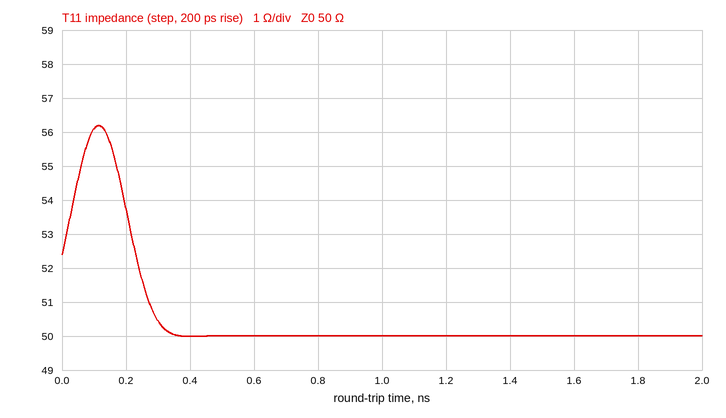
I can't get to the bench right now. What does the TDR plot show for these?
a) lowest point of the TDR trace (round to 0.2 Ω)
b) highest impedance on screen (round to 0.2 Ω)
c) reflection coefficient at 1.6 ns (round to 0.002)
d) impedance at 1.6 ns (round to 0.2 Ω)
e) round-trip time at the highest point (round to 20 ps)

50.0 Ω
56.2 Ω
0.000
50.0 Ω
120 ps
